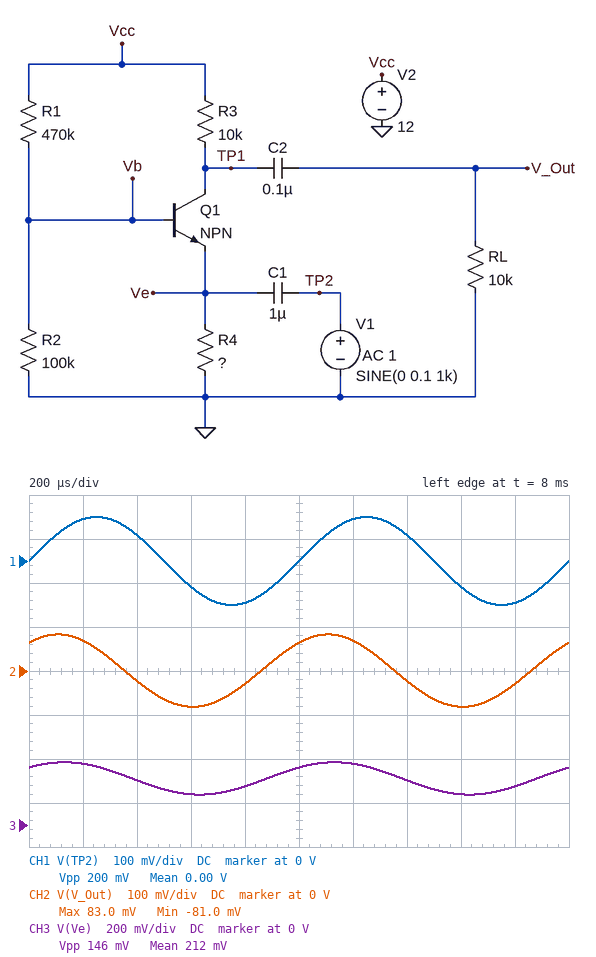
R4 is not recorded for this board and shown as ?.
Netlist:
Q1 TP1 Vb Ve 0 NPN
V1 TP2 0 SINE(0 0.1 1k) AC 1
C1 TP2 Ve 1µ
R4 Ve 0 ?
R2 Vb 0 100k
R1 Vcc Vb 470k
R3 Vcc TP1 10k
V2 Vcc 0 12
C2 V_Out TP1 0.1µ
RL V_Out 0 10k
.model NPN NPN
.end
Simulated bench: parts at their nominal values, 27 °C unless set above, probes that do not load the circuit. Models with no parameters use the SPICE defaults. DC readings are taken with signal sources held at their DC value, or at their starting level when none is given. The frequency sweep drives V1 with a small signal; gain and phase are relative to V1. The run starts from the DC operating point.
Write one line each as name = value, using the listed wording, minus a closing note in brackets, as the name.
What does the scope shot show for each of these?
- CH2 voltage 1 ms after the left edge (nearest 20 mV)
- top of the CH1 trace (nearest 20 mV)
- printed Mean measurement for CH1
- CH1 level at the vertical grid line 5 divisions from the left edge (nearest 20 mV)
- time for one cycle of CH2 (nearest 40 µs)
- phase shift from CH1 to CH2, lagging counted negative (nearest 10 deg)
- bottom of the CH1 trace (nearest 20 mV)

CH2 voltage 1 ms after the left edge = 60 mV
top of the CH1 trace = 100 mV
printed Mean measurement for CH1 = 0.00 V
CH1 level at the vertical grid line 5 divisions from the left edge = 0 V
time for one cycle of CH2 = 1.00 ms
phase shift from CH1 to CH2, lagging counted negative = 50 deg
bottom of the CH1 trace = -100 mV
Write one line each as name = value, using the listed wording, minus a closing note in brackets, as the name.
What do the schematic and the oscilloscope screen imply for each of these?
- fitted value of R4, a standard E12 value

fitted value of R4, a standard E12 value = 180 Ω
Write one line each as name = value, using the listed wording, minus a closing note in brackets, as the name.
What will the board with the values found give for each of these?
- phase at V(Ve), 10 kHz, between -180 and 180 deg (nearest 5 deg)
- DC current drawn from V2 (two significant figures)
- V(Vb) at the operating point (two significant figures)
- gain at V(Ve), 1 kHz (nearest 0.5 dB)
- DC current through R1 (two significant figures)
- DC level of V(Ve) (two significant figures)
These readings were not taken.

phase at V(Ve), 10 kHz, between -180 and 180 deg = 5 deg
DC current drawn from V2 = 1.2 mA
V(Vb) at the operating point = 990 mV
gain at V(Ve), 1 kHz = -2.5 dB
DC current through R1 = 23 µA
DC level of V(Ve) = 210 mV
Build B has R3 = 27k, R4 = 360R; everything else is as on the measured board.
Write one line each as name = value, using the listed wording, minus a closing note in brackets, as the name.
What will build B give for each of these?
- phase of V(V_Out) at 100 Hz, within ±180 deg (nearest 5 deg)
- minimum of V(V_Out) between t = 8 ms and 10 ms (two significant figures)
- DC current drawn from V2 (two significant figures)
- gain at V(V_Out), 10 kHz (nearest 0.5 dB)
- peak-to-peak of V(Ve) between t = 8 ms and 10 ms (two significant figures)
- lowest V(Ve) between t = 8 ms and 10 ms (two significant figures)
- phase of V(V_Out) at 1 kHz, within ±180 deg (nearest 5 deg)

phase of V(V_Out) at 100 Hz, within ±180 deg = 135 deg
minimum of V(V_Out) between t = 8 ms and 10 ms = -91 mV
DC current drawn from V2 = 460 µA
gain at V(V_Out), 10 kHz = 0 dB
peak-to-peak of V(Ve) between t = 8 ms and 10 ms = 180 mV
lowest V(Ve) between t = 8 ms and 10 ms = 71 mV
phase of V(V_Out) at 1 kHz, within ±180 deg = 35 deg
